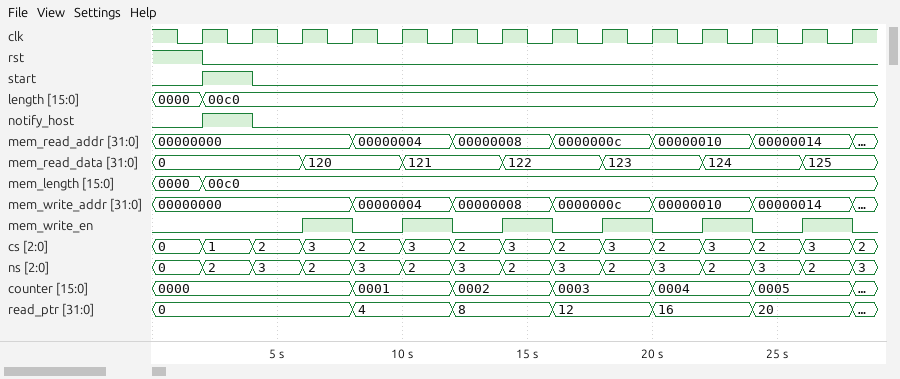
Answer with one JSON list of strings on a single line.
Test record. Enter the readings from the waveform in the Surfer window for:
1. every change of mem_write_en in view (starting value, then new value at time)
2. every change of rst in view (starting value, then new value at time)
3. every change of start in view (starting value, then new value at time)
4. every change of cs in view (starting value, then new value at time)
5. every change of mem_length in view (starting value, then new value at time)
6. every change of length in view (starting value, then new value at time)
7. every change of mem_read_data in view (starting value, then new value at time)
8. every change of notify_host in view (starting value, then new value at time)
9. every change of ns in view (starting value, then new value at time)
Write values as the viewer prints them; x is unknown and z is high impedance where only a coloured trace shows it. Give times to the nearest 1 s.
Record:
["0, 1 at 6 s, 0 at 8 s, 1 at 10 s, 0 at 12 s, 1 at 14 s, 0 at 16 s, 1 at 18 s, 0 at 20 s, 1 at 22 s, 0 at 24 s, 1 at 26 s, 0 at 28 s", "1, 0 at 2 s", "0, 1 at 2 s, 0 at 4 s", "0, 1 at 2 s, 2 at 4 s, 3 at 6 s, 2 at 8 s, 3 at 10 s, 2 at 12 s, 3 at 14 s, 2 at 16 s, 3 at 18 s, 2 at 20 s, 3 at 22 s, 2 at 24 s, 3 at 26 s, 2 at 28 s", "0000, 00c0 at 2 s", "0000, 00c0 at 2 s", "0, 120 at 6 s, 121 at 10 s, 122 at 14 s, 123 at 18 s, 124 at 22 s, 125 at 26 s", "0, 1 at 2 s, 0 at 4 s", "0, 2 at 2 s, 3 at 4 s, 2 at 6 s, 3 at 8 s, 2 at 10 s, 3 at 12 s, 2 at 14 s, 3 at 16 s, 2 at 18 s, 3 at 20 s, 2 at 22 s, 3 at 24 s, 2 at 26 s, 3 at 28 s"]
